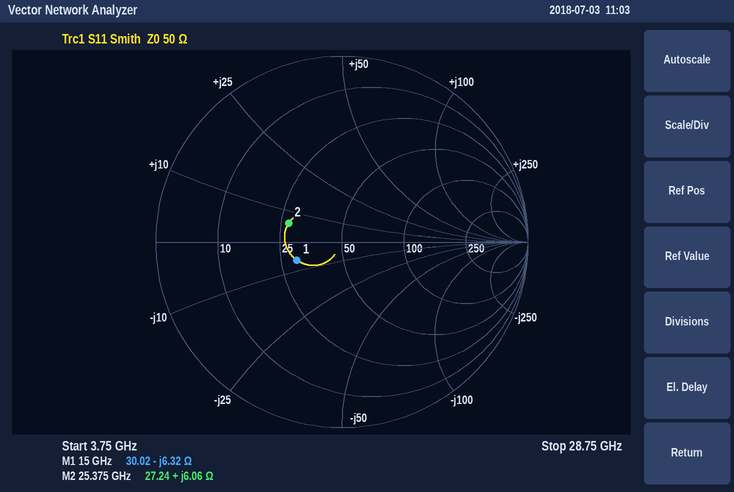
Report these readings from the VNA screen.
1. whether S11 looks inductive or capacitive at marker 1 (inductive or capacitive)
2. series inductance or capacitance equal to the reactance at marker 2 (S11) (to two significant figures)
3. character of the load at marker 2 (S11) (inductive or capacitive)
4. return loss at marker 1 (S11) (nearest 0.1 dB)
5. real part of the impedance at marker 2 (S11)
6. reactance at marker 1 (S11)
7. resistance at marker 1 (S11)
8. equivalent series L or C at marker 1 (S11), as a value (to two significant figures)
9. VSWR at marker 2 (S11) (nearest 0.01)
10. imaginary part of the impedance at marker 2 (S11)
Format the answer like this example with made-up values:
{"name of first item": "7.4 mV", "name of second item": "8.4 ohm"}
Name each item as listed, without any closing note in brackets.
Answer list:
{"whether S11 looks inductive or capacitive at marker 1": "capacitive", "series inductance or capacitance equal to the reactance at marker 2 (S11)": "38 pH", "character of the load at marker 2 (S11)": "inductive", "return loss at marker 1 (S11)": "11.7 dB", "real part of the impedance at marker 2": "27.24 Ω", "reactance at marker 1": "-6.32 Ω", "resistance at marker 1": "30.02 Ω", "equivalent series L or C at marker 1 (S11), as a value": "1.7 pF", "VSWR at marker 2 (S11)": "1.87", "imaginary part of the impedance at marker 2": "+6.06 Ω"}
